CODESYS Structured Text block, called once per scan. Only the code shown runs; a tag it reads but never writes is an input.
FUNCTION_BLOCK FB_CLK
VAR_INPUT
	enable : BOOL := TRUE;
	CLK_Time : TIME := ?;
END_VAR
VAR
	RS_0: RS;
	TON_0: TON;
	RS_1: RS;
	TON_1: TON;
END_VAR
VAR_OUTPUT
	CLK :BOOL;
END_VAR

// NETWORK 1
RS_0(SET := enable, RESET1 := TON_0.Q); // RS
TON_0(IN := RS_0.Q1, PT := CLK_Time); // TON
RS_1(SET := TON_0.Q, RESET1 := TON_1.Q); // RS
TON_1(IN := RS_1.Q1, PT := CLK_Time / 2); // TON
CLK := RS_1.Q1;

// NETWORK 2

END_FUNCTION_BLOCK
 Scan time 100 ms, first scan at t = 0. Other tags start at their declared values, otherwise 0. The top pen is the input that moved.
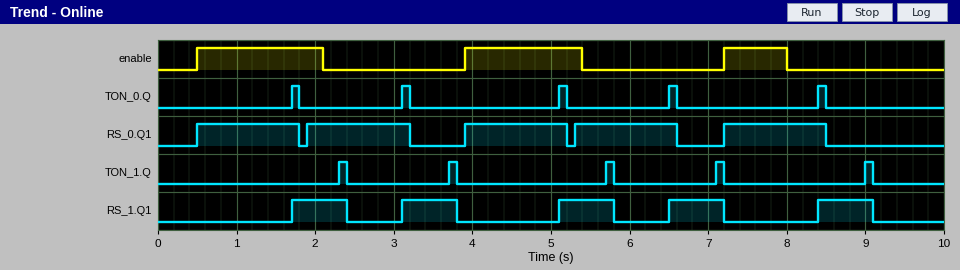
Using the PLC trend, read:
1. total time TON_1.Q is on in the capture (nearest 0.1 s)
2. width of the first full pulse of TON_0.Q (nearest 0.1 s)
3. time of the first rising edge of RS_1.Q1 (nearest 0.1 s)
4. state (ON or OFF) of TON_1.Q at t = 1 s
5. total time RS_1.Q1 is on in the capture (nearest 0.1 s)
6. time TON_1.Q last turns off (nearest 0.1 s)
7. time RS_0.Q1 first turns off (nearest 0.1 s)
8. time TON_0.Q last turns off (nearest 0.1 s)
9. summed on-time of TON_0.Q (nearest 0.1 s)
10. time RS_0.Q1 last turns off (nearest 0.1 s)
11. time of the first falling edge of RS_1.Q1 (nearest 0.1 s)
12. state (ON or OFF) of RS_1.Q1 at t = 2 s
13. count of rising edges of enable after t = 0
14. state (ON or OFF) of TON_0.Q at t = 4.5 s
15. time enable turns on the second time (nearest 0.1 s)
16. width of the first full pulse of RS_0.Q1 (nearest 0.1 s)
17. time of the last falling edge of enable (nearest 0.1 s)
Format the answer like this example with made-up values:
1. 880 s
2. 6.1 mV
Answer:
1. 0.5 s
2. 0.1 s
3. 1.7 s
4. OFF
5. 3.5 s
6. 9.1 s
7. 1.8 s
8. 8.5 s
9. 0.5 s
10. 8.5 s
11. 2.4 s
12. ON
13. 3
14. OFF
15. 3.9 s
16. 1.3 s
17. 8.0 s
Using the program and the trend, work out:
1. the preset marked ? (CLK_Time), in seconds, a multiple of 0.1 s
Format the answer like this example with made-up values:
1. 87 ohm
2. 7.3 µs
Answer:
1. 1.2 s
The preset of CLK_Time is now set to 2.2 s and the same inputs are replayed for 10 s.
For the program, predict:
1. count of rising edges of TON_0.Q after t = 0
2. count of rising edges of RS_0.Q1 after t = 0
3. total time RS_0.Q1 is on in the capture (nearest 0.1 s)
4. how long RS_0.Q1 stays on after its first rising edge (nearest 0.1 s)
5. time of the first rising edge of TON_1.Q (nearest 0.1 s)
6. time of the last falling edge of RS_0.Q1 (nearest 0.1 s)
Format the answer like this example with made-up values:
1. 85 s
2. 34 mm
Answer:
1. 3
2. 3
3. 6.9 s
4. 2.3 s
5. 3.8 s
6. 9.5 s
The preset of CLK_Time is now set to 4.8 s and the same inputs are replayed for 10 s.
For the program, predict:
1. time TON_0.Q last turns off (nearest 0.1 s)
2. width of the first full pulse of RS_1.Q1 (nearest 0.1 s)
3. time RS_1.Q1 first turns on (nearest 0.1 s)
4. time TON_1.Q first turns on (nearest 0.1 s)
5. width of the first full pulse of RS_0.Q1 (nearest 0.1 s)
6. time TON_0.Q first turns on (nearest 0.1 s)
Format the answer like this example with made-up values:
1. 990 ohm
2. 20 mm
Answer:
1. 5.4 s
2. 2.5 s
3. 5.3 s
4. 7.7 s
5. 4.9 s
6. 5.3 s
